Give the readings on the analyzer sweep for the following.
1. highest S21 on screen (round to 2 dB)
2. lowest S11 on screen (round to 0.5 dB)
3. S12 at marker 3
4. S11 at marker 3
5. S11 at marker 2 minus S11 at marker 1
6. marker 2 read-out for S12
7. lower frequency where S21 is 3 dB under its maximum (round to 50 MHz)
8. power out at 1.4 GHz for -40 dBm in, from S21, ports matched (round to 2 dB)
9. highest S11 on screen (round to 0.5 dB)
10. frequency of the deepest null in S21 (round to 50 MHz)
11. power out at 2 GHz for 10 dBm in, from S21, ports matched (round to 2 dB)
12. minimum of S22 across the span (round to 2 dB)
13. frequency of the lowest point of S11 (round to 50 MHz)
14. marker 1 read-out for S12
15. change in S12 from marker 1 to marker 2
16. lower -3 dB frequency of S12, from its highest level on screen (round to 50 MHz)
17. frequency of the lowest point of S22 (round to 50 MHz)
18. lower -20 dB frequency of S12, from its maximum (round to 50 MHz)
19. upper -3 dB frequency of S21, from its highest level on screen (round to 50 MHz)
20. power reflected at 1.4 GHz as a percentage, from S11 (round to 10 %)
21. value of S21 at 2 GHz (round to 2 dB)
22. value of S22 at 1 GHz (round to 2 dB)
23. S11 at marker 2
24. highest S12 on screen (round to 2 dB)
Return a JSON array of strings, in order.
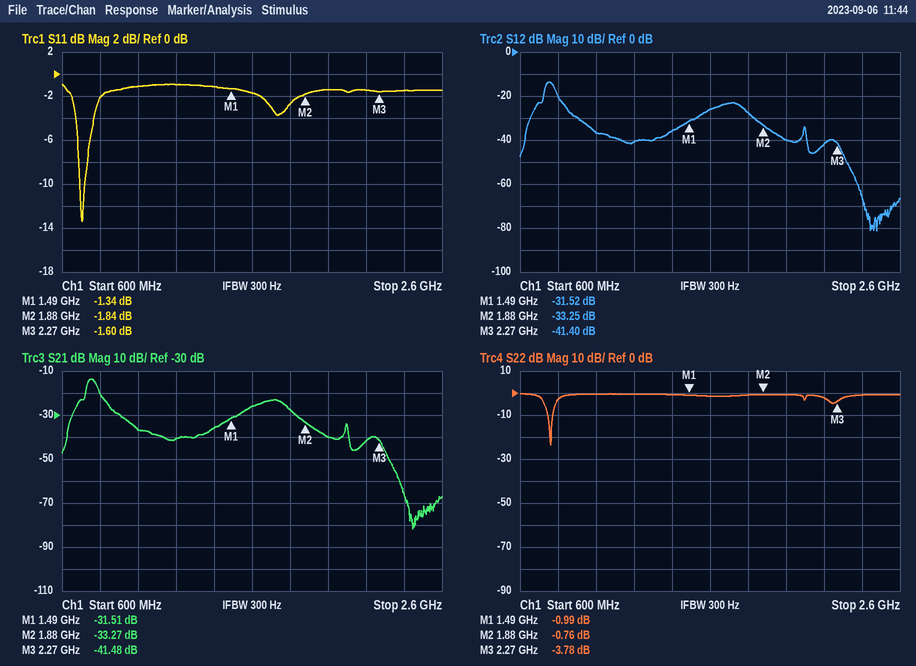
["-14 dB", "-13.5 dB", "-41.40 dB", "-1.60 dB", "-0.50 dB", "-33.25 dB", "750 MHz", "-76 dBm", "-1.0 dB", "2.45 GHz", "-30 dBm", "-24 dB", "700 MHz", "-31.52 dB", "-1.73 dB", "750 MHz", "750 MHz", "650 MHz", "800 MHz", "80 %", "-40 dB", "0 dB", "-1.84 dB", "-14 dB"]
